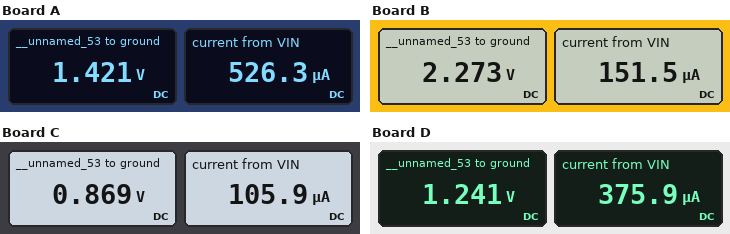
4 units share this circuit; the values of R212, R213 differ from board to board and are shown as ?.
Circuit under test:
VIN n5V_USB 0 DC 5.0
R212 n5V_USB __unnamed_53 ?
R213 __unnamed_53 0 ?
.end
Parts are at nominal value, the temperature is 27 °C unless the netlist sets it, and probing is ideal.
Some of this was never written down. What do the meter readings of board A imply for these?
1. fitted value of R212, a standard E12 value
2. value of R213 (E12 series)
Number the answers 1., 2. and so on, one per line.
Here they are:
1. 6.8 kΩ
2. 2.7 kΩ
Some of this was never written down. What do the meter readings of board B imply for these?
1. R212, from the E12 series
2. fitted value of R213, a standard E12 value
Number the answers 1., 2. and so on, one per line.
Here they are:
1. 18 kΩ
2. 15 kΩ
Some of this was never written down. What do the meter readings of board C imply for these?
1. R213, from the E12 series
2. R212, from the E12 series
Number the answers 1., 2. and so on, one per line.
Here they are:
1. 8.2 kΩ
2. 39 kΩ
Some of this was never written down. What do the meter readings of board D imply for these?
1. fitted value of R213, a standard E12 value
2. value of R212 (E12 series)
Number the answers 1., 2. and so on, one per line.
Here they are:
1. 3.3 kΩ
2. 10 kΩ
